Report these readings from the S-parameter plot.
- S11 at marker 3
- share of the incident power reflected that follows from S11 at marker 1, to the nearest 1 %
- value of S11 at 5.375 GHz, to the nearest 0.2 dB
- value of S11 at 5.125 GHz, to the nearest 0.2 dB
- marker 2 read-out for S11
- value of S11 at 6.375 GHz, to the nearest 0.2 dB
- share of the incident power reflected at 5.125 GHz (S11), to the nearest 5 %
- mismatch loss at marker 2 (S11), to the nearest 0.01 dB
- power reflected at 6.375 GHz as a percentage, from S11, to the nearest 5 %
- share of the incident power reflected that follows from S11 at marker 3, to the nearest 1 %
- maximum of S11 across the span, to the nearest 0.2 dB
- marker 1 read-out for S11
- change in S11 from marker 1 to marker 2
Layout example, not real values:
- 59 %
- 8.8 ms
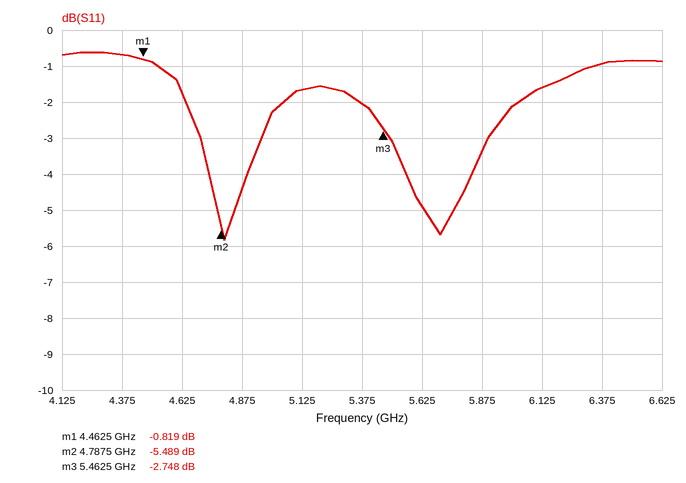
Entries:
- -2.748 dB
- 83 %
- -2.0 dB
- -1.6 dB
- -5.489 dB
- -1.0 dB
- 70 %
- 1.44 dB
- 80 %
- 53 %
- -0.6 dB
- -0.819 dB
- -4.670 dB
